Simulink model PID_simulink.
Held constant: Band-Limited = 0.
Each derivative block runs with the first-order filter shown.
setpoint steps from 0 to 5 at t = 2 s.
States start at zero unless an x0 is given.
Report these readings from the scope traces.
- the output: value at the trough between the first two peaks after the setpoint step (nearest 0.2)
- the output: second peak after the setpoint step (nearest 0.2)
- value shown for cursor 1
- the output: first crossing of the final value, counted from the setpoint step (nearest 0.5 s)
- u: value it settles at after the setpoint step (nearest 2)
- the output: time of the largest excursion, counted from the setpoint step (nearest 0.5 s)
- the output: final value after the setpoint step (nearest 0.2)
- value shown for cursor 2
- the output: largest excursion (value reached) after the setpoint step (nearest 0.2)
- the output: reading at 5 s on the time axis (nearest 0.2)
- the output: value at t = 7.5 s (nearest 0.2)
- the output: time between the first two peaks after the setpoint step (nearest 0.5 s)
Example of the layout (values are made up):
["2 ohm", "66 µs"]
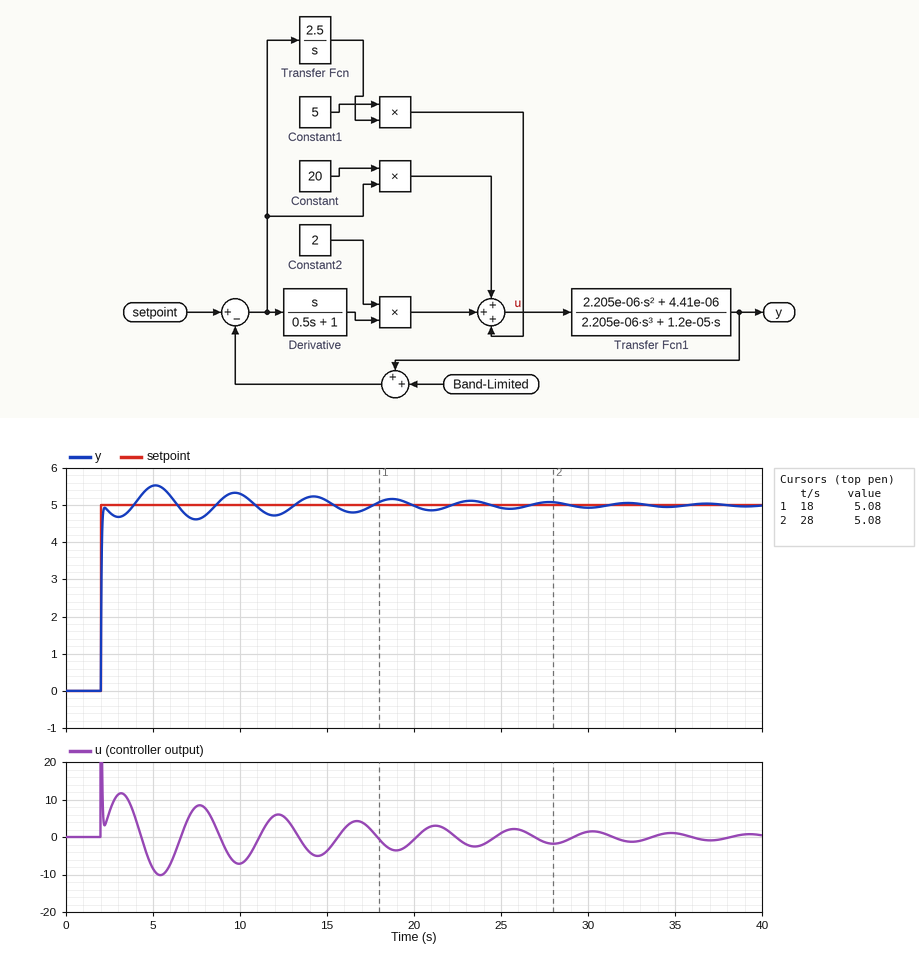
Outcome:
["4.6", "5.4", "5.08", "2.0 s", "0", "3.0 s", "5.0", "5.08", "5.6", "5.6", "4.6", "4.5 s"]
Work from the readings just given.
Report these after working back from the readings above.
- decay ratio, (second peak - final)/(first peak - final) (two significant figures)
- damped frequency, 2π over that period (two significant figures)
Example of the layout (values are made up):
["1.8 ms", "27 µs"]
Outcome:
["0.67", "1.4 rad/s"]
